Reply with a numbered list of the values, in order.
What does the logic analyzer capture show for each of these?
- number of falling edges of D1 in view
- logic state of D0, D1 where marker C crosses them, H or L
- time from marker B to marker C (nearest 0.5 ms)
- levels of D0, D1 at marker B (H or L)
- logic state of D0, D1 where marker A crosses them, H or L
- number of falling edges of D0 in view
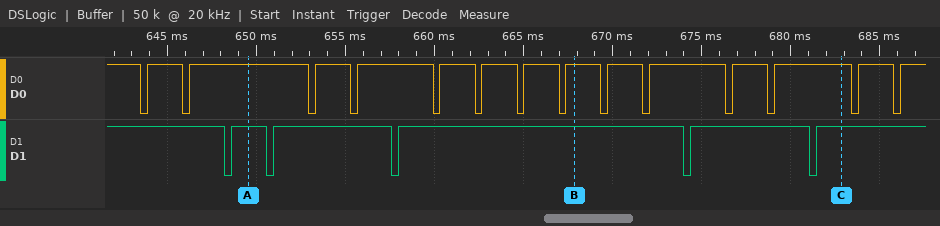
1. 5
2. D0=H, D1=H
3. 15 ms
4. D0=H, D1=H
5. D0=H, D1=H
6. 14
